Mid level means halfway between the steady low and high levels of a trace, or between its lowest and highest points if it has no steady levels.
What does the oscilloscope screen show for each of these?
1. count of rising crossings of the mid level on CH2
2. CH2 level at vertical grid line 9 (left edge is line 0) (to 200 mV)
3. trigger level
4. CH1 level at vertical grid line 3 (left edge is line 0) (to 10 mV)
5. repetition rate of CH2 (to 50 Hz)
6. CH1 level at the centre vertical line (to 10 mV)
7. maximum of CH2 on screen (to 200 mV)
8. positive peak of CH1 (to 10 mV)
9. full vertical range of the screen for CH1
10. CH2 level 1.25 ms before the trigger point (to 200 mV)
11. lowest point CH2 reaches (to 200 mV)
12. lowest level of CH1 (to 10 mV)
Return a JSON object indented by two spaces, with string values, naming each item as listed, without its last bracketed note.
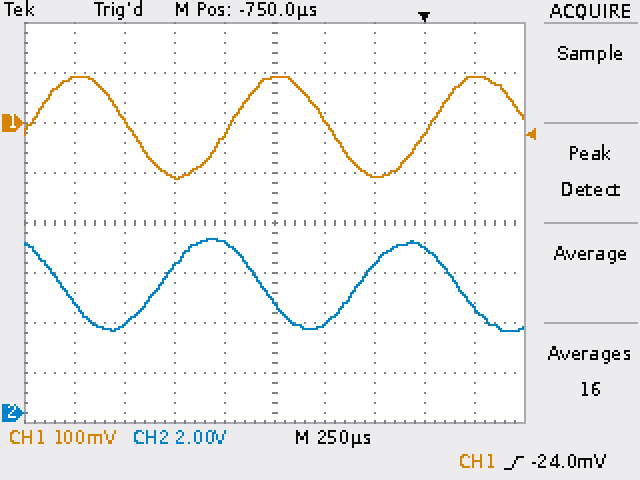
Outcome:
{
  "count of rising crossings of the mid level on CH2": "2",
  "CH2 level at vertical grid line 9 (left edge is line 0)": "4.2 V",
  "trigger level": "-24.0 mV",
  "CH1 level at vertical grid line 3 (left edge is line 0)": "-110 mV",
  "repetition rate of CH2": "1.00 kHz",
  "CH1 level at the centre vertical line": "90 mV",
  "maximum of CH2 on screen": "7.0 V",
  "positive peak of CH1": "90 mV",
  "full vertical range of the screen for CH1": "800 mV",
  "CH2 level 1.25 ms before the trigger point": "5.8 V",
  "lowest point CH2 reaches": "3.2 V",
  "lowest level of CH1": "-110 mV"
}
